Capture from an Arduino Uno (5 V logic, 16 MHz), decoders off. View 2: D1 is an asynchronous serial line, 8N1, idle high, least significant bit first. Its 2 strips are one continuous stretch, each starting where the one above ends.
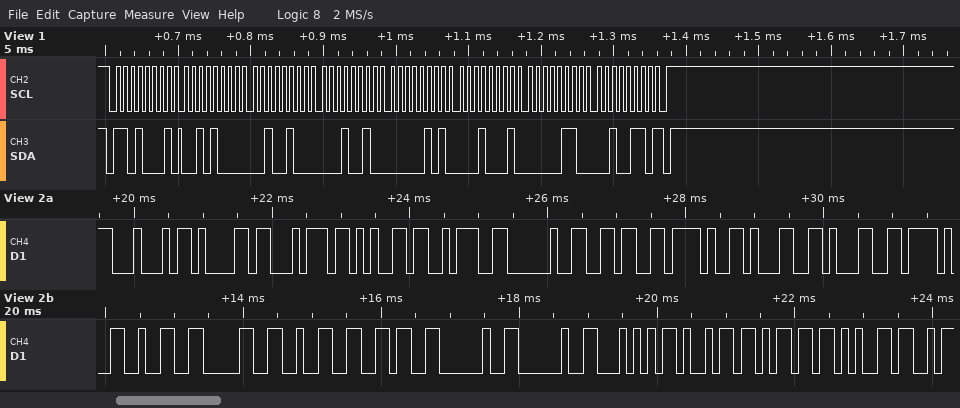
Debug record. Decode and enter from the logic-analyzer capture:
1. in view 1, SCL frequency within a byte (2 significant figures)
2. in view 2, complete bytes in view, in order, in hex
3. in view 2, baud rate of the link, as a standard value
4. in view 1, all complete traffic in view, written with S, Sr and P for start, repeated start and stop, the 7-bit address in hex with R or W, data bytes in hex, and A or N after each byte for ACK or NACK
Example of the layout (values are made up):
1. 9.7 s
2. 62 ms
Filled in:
1. 100 kHz
2. 44 61 74 65 3A 20 36 2F 31 31 2F 32 30 32 36 20 20 54 69 6D 65
3. 9600 baud
4. S 68R A 28 A 24 A 12 A 05 A 11 A 06 A 26 N P
